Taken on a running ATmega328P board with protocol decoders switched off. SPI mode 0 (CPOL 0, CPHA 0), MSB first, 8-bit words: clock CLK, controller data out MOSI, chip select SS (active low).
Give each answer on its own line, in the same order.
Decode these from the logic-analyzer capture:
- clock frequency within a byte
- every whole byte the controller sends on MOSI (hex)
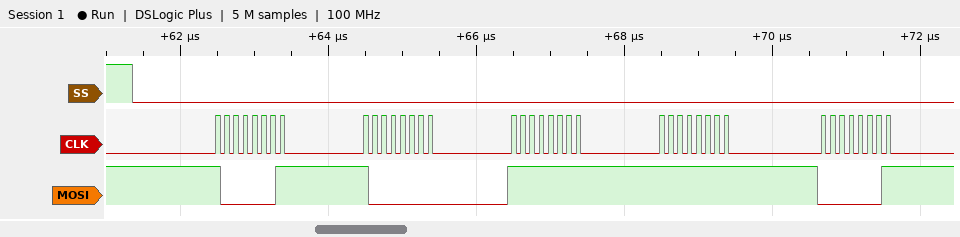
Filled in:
8 MHz
81 80 FF FF 01
